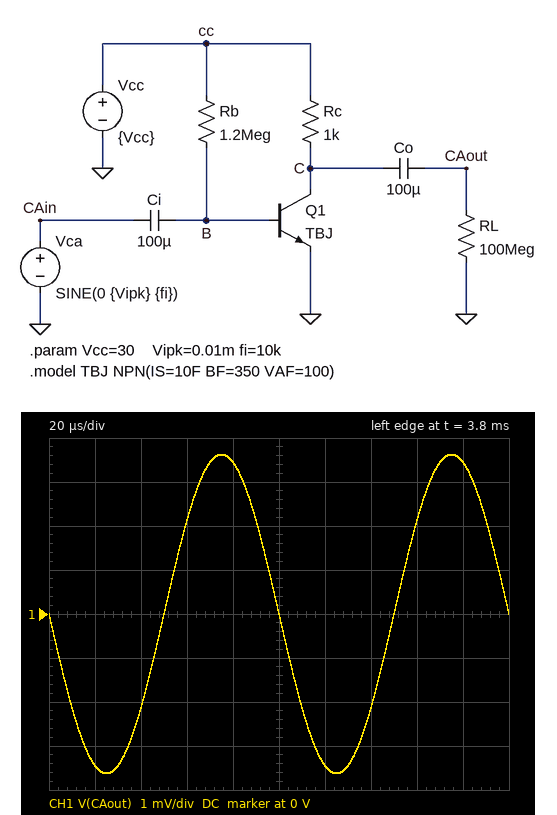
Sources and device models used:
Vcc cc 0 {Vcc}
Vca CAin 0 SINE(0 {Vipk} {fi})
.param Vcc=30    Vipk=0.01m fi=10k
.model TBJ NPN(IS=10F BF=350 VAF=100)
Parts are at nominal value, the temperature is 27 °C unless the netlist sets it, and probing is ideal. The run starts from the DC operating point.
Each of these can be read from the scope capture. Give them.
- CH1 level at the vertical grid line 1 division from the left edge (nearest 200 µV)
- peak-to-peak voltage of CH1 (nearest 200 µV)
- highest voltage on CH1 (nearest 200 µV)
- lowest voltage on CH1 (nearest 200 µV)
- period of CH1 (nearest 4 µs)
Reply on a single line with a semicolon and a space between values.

-3.4 mV; 7.2 mV; 3.6 mV; -3.6 mV; 100 µs
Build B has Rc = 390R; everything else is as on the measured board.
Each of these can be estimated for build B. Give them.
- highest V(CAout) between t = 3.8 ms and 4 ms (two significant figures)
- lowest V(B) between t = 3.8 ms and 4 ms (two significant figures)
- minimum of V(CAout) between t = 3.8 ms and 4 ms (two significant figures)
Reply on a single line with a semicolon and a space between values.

1.6 mV; 710 mV; -1.6 mV
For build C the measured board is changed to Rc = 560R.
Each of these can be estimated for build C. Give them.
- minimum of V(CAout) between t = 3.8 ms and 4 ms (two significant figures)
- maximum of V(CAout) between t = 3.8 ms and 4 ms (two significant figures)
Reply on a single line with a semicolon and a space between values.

-2.2 mV; 2.2 mV
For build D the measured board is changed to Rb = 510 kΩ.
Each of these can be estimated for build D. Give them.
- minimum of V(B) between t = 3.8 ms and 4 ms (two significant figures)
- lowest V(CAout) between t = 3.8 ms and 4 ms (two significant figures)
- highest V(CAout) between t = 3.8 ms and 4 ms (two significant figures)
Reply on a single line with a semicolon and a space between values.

730 mV; -7.0 mV; 7.0 mV
